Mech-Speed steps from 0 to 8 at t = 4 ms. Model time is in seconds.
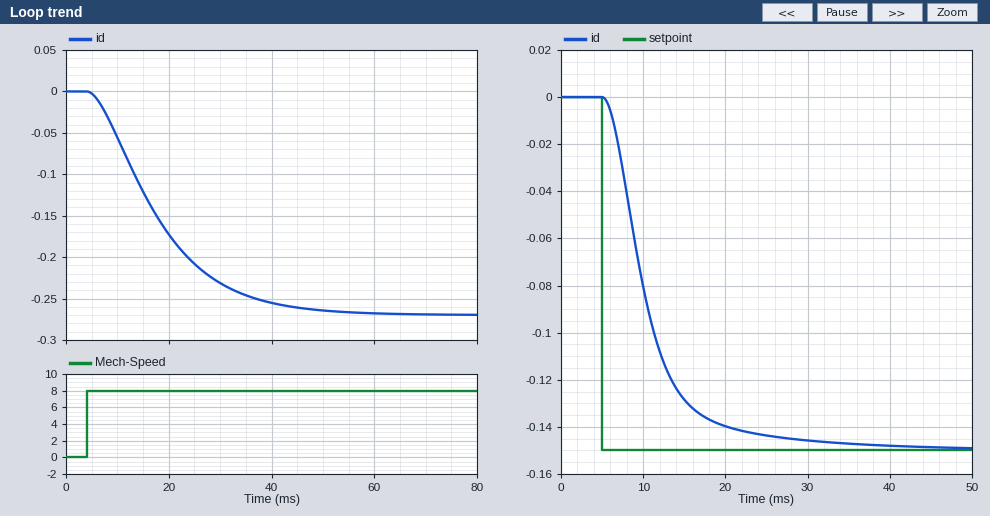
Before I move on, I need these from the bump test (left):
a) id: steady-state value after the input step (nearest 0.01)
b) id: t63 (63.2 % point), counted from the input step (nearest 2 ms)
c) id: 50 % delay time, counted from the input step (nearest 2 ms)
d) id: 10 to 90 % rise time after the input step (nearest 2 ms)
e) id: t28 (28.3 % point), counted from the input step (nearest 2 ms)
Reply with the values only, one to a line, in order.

-0.27
16 ms
12 ms
26 ms
8 ms
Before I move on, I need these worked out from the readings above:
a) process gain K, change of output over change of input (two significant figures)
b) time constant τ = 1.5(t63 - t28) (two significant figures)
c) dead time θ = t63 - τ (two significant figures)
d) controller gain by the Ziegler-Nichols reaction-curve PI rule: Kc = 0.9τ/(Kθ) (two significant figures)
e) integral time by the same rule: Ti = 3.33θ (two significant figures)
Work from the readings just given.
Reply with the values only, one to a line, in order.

-0.034
12 ms
4.0 ms
-79
13 ms
